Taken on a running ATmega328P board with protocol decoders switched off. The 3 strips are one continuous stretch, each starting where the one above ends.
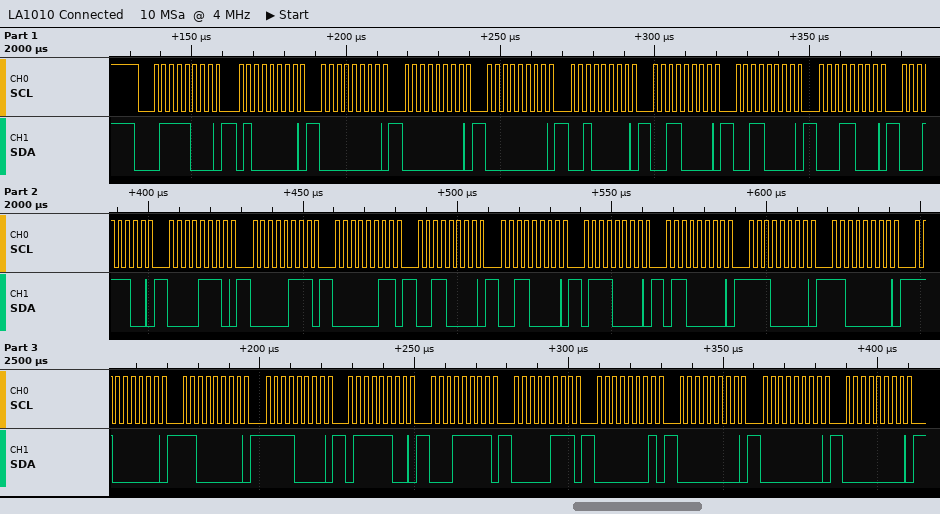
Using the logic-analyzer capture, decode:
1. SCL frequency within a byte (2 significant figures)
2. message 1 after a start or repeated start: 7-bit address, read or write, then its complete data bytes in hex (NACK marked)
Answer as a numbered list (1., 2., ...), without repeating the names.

1. 400 kHz
2. 0x3C write: 40 00 00 00 20 30 30 18 1C 0E 07 03 30 30 70 60 E0 C0 C0 C0 F0 7C 1F 07 01 00 00 00
